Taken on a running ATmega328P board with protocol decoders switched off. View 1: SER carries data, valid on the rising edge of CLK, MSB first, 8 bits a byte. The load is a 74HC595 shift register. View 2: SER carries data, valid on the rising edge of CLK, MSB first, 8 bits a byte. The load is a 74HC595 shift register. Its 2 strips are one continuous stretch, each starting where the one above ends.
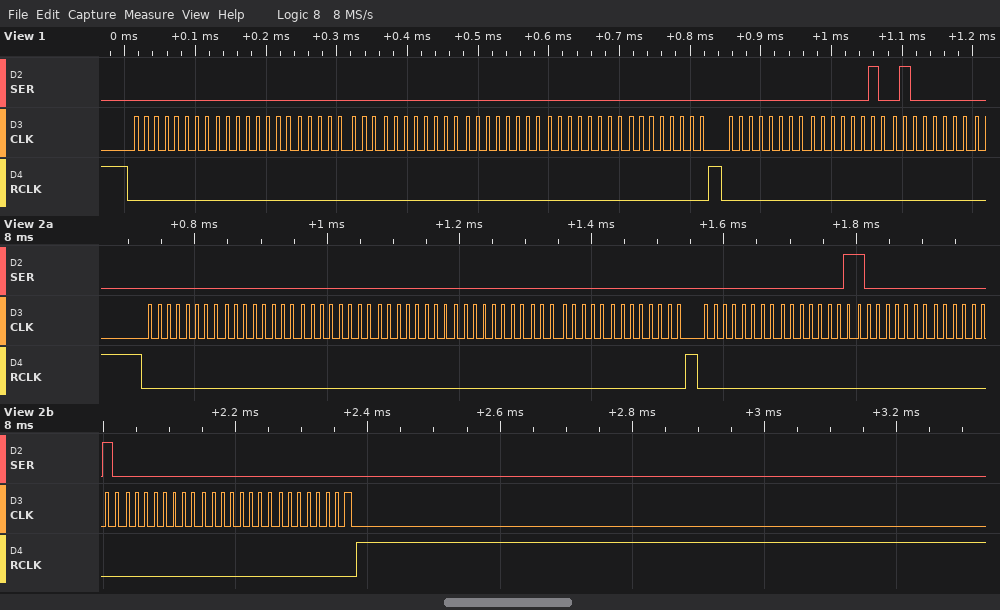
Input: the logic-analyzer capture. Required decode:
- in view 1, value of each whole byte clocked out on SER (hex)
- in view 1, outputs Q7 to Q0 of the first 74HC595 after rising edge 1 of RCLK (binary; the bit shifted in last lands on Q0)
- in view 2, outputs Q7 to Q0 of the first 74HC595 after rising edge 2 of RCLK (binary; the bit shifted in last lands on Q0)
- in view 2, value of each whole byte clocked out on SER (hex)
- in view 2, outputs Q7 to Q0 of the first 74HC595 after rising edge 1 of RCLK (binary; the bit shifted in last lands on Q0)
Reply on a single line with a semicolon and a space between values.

0x00 0x00 0x00 0x00 0x00 0x00 0x00 0x00 0x02 0x40; 00000000; 00000000; 00 00 00 00 00 00 00 00 01 80 02 00 00 00; 00000000
